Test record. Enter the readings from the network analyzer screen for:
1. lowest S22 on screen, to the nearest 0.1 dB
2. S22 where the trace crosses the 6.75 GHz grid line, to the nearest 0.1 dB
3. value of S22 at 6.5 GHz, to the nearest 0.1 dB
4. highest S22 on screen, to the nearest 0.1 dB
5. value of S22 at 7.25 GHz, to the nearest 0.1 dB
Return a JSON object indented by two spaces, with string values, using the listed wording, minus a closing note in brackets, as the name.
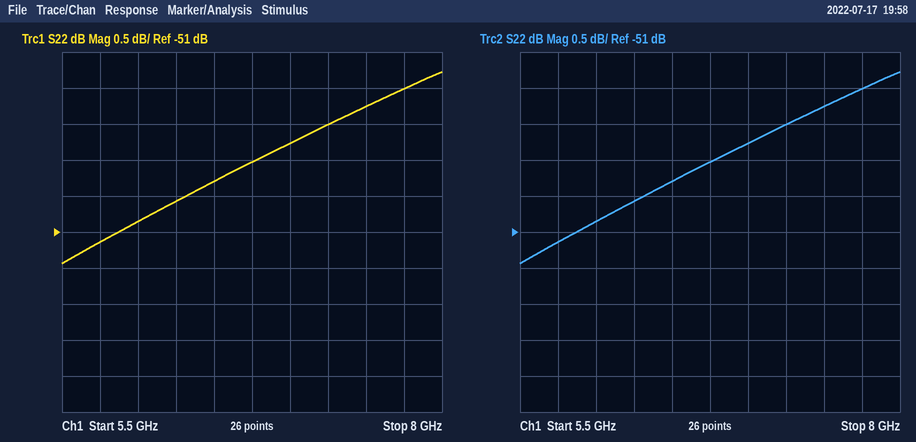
{
  "lowest S22 on screen, to the nearest 0.1 dB": "-51.4 dB",
  "S22 where the trace crosses the 6.75 GHz grid line, to the nearest 0.1 dB": "-50.0 dB",
  "value of S22 at 6.5 GHz, to the nearest 0.1 dB": "-50.3 dB",
  "highest S22 on screen, to the nearest 0.1 dB": "-48.8 dB",
  "value of S22 at 7.25 GHz, to the nearest 0.1 dB": "-49.5 dB"
}
